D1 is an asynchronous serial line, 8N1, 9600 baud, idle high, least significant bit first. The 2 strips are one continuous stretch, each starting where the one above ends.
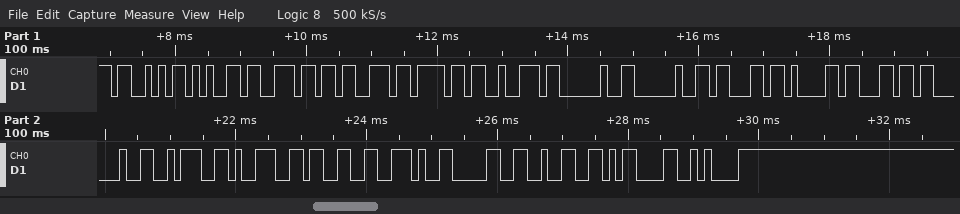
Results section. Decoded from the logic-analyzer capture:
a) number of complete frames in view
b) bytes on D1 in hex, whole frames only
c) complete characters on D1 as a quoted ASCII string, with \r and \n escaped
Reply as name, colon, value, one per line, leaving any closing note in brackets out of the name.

number of complete frames in view: 20
bytes on D1 in hex, whole frames only: 53 65 6E 73 6F 72 20 20 63 61 6C 20 3A 39 33 2E 30 32 0D 0A
complete characters on D1 as a quoted ASCII string, with \r and \n escaped: "Sensor  cal :93.02\r\n"
